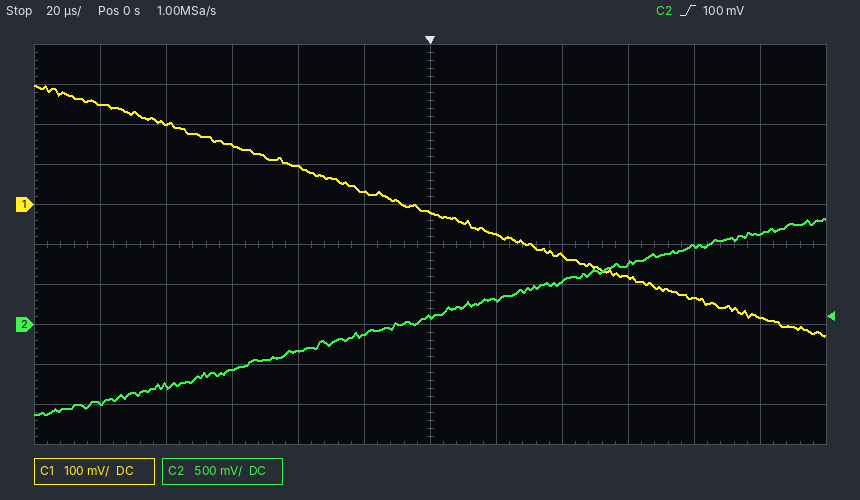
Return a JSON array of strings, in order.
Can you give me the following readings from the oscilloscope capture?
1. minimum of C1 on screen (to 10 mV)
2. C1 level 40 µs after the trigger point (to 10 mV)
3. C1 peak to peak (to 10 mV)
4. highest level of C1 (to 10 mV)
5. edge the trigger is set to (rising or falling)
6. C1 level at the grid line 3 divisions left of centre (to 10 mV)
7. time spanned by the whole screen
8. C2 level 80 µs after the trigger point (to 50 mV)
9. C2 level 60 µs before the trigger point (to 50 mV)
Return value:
["-330 mV", "-130 mV", "630 mV", "300 mV", "rising", "150 mV", "240 µs", "1.00 V", "-550 mV"]
